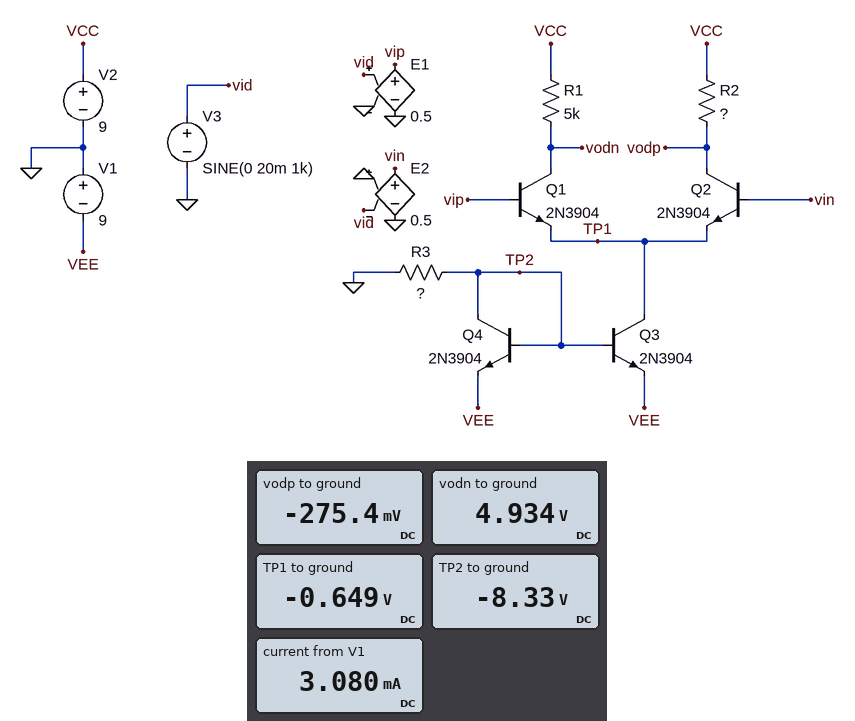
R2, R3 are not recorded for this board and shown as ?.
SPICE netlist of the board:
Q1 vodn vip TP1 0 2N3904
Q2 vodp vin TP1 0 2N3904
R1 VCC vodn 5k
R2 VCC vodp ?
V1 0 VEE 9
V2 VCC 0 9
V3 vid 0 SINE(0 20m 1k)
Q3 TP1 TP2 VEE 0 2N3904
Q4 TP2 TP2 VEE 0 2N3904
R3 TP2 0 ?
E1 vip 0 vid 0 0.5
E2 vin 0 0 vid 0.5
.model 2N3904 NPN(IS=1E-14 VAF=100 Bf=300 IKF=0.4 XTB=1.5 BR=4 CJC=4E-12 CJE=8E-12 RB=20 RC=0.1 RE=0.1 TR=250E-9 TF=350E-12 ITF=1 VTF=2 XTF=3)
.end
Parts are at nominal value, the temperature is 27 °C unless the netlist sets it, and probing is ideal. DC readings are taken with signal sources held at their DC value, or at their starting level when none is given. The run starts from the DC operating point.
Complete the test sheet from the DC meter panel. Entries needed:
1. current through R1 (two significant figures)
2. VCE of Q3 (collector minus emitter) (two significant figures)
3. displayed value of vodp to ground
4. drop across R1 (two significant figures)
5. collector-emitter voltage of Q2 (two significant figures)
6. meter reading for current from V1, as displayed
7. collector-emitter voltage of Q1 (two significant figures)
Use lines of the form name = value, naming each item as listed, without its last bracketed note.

current through R1 = 810 µA
VCE of Q3 (collector minus emitter) = 8.4 V
displayed value of vodp to ground = -275.4 mV
drop across R1 = 4.1 V
collector-emitter voltage of Q2 = 370 mV
meter reading for current from V1, as displayed = 3.080 mA
collector-emitter voltage of Q1 = 5.6 V
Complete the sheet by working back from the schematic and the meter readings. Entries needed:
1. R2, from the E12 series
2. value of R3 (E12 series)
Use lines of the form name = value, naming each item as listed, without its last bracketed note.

R2, from the E12 series = 12 kΩ
value of R3 = 5.6 kΩ
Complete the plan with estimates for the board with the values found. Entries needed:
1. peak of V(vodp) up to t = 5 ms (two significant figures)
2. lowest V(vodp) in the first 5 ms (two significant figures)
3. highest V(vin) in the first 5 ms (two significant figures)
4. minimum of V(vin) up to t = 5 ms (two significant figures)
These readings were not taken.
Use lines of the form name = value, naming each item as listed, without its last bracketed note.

peak of V(vodp) up to t = 5 ms = 3.0 V
lowest V(vodp) in the first 5 ms = -620 mV
highest V(vin) in the first 5 ms = 10 mV
minimum of V(vin) up to t = 5 ms = -10 mV
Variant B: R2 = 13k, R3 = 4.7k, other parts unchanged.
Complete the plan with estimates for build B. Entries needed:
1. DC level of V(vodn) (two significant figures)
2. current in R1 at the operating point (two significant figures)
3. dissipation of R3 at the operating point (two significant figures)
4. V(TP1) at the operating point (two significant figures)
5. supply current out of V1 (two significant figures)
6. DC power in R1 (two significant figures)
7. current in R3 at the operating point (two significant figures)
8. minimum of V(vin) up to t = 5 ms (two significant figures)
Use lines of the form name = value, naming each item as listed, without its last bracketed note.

DC level of V(vodn) = 3.5 V
current in R1 at the operating point = 1.1 mA
dissipation of R3 at the operating point = 15 mW
V(TP1) at the operating point = -660 mV
supply current out of V1 = 3.7 mA
DC power in R1 = 6.0 mW
current in R3 at the operating point = 1.8 mA
minimum of V(vin) up to t = 5 ms = -10 mV
